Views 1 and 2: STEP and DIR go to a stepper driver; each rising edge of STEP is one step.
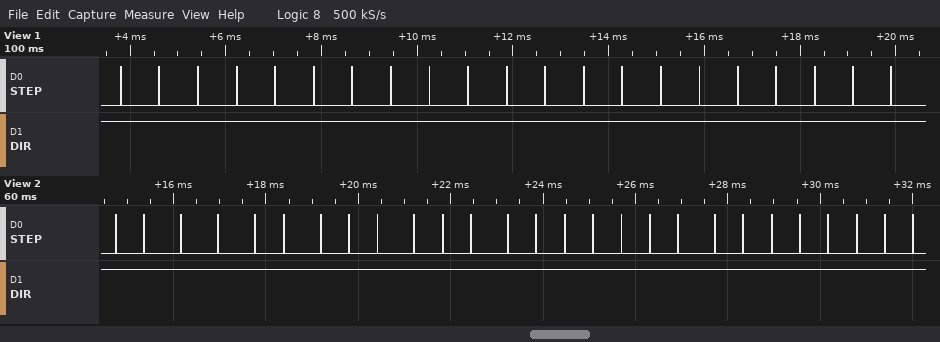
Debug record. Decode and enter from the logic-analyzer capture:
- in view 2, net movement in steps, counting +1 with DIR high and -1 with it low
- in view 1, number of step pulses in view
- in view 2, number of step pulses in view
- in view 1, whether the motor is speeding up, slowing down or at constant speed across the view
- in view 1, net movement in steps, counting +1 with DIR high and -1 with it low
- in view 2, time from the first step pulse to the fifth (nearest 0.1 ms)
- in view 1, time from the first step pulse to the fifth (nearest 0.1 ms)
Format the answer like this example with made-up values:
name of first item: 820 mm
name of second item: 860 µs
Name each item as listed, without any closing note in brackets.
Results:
in view 2, net movement in steps, counting +1 with DIR high and -1 with it low: +27
in view 1, number of step pulses in view: 21
in view 2, number of step pulses in view: 27
in view 1, whether the motor is speeding up, slowing down or at constant speed across the view: constant speed
in view 1, net movement in steps, counting +1 with DIR high and -1 with it low: +21
in view 2, time from the first step pulse to the fifth: 3.0 ms
in view 1, time from the first step pulse to the fifth: 3.2 ms
